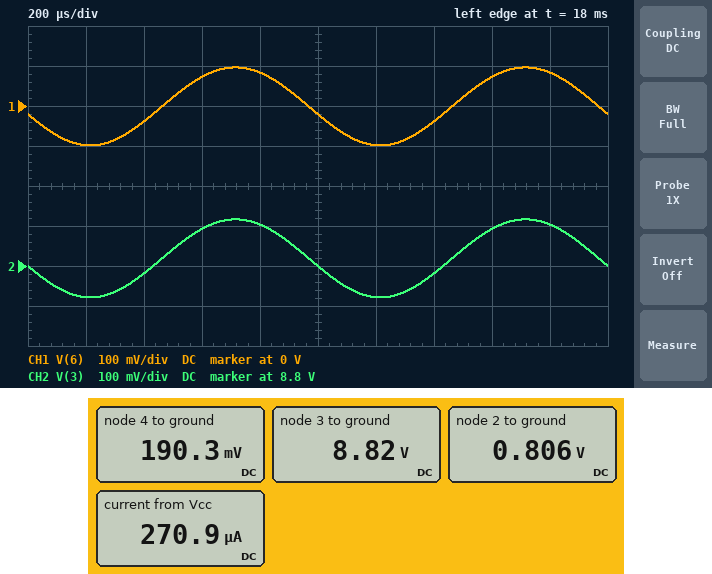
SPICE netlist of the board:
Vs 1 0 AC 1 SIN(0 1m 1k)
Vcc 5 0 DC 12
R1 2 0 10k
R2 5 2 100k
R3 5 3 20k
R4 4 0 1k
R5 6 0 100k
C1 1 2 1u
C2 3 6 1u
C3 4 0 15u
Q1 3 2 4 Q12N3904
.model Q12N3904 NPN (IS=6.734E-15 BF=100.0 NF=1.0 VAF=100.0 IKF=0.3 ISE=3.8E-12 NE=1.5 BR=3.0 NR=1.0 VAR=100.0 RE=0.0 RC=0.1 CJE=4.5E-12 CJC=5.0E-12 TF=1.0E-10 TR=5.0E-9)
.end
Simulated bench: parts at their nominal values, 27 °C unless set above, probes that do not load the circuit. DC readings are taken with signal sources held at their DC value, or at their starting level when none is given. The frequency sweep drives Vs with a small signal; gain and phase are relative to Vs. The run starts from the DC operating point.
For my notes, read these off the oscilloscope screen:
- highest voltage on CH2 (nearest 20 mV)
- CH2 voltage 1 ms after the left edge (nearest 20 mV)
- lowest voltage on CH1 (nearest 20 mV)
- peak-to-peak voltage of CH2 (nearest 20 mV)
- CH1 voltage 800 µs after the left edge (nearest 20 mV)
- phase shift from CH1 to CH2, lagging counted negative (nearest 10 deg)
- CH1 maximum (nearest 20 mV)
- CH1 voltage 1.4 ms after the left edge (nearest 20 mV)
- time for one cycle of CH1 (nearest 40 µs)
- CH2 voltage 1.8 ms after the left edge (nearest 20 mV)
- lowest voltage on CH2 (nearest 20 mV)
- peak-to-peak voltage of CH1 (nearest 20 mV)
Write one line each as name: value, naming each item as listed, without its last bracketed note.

highest voltage on CH2: 8.92 V
CH2 voltage 1 ms after the left edge: 8.80 V
lowest voltage on CH1: -100 mV
peak-to-peak voltage of CH2: 200 mV
CH1 voltage 800 µs after the left edge: 80 mV
phase shift from CH1 to CH2, lagging counted negative: 0 deg
CH1 maximum: 100 mV
CH1 voltage 1.4 ms after the left edge: -40 mV
time for one cycle of CH1: 1.00 ms
CH2 voltage 1.8 ms after the left edge: 8.90 V
lowest voltage on CH2: 8.72 V
peak-to-peak voltage of CH1: 200 mV
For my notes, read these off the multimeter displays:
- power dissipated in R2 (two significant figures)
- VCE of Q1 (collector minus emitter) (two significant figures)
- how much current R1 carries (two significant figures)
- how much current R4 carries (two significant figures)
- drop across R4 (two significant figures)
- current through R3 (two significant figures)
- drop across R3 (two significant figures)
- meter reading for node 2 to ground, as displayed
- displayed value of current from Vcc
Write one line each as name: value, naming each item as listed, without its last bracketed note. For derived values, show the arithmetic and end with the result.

power dissipated in R2: (12 V - 806 mV)^2 / 100 kΩ = 1.3 mW
VCE of Q1 (collector minus emitter): 8.82 V - 190.3 mV = 8.6 V
how much current R1 carries: (806 mV) / 10 kΩ = 81 µA
how much current R4 carries: (190.3 mV) / 1 kΩ = 190 µA
drop across R4: 190.3 mV = 190 mV
current through R3: (12 V - 8.82 V) / 20 kΩ = 160 µA
drop across R3: 12 V - 8.82 V = 3.2 V
meter reading for node 2 to ground, as displayed: 0.806 V
displayed value of current from Vcc: 270.9 µA
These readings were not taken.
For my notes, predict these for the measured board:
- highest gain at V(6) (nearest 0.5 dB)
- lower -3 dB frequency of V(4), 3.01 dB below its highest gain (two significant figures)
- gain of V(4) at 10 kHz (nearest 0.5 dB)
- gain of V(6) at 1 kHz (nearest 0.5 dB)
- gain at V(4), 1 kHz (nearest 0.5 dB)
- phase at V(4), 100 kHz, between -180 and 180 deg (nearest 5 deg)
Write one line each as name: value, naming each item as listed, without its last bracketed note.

highest gain at V(6): 40.0 dB
lower -3 dB frequency of V(4), 3.01 dB below its highest gain: 12 Hz
gain of V(4) at 10 kHz: -43.0 dB
gain of V(6) at 1 kHz: 40.0 dB
gain at V(4), 1 kHz: -23.0 dB
phase at V(4), 100 kHz, between -180 and 180 deg: -90 deg
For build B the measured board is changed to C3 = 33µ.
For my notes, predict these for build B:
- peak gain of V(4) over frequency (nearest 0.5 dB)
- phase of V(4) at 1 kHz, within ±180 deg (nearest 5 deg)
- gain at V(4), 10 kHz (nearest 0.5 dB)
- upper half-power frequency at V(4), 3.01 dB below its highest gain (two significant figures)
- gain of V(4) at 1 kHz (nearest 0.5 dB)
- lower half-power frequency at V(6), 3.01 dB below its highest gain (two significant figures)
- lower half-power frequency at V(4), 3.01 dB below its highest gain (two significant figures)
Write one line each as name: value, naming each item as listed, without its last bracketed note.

peak gain of V(4) over frequency: -15.0 dB
phase of V(4) at 1 kHz, within ±180 deg: -80 deg
gain at V(4), 10 kHz: -49.5 dB
upper half-power frequency at V(4), 3.01 dB below its highest gain: 190 Hz
gain of V(4) at 1 kHz: -30.0 dB
lower half-power frequency at V(6), 3.01 dB below its highest gain: 180 Hz
lower half-power frequency at V(4), 3.01 dB below its highest gain: 6.7 Hz
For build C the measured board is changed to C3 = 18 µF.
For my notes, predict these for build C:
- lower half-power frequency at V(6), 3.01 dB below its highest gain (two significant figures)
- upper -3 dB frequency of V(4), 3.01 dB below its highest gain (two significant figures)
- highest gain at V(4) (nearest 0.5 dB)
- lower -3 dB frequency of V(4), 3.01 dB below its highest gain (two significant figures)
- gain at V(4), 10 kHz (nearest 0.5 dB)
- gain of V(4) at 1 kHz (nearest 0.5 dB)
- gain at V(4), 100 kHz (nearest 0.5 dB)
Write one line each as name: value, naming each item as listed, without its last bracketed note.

lower half-power frequency at V(6), 3.01 dB below its highest gain: 210 Hz
upper -3 dB frequency of V(4), 3.01 dB below its highest gain: 230 Hz
highest gain at V(4): -11.0 dB
lower -3 dB frequency of V(4), 3.01 dB below its highest gain: 10 Hz
gain at V(4), 10 kHz: -44.5 dB
gain of V(4) at 1 kHz: -24.5 dB
gain at V(4), 100 kHz: -64.5 dB
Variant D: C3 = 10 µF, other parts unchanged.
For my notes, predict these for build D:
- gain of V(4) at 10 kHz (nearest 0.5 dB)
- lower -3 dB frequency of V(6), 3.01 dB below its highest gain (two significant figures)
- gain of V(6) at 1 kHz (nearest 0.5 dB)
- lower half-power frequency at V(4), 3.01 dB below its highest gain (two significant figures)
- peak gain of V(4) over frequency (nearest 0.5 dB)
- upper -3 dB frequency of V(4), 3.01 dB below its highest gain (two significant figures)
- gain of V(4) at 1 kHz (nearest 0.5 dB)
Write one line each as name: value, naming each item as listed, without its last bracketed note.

gain of V(4) at 10 kHz: -39.5 dB
lower -3 dB frequency of V(6), 3.01 dB below its highest gain: 260 Hz
gain of V(6) at 1 kHz: 39.5 dB
lower half-power frequency at V(4), 3.01 dB below its highest gain: 15 Hz
peak gain of V(4) over frequency: -8.0 dB
upper -3 dB frequency of V(4), 3.01 dB below its highest gain: 290 Hz
gain of V(4) at 1 kHz: -19.5 dB
